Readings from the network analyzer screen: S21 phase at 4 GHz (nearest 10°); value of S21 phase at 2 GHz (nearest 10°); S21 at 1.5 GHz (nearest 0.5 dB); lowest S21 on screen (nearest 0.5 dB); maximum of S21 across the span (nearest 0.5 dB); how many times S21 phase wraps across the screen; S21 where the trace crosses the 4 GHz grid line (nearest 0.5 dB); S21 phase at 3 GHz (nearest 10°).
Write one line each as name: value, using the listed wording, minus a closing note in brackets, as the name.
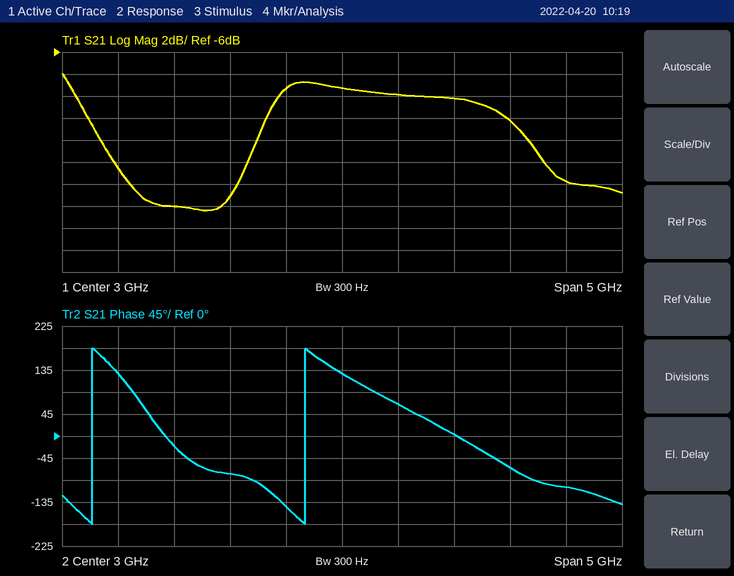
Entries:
S21 phase at 4 GHz: 0°
value of S21 phase at 2 GHz: -80°
S21 at 1.5 GHz: -20.0 dB
lowest S21 on screen: -20.5 dB
maximum of S21 across the span: -8.0 dB
how many times S21 phase wraps across the screen: 2
S21 where the trace crosses the 4 GHz grid line: -10.0 dB
S21 phase at 3 GHz: 130°
